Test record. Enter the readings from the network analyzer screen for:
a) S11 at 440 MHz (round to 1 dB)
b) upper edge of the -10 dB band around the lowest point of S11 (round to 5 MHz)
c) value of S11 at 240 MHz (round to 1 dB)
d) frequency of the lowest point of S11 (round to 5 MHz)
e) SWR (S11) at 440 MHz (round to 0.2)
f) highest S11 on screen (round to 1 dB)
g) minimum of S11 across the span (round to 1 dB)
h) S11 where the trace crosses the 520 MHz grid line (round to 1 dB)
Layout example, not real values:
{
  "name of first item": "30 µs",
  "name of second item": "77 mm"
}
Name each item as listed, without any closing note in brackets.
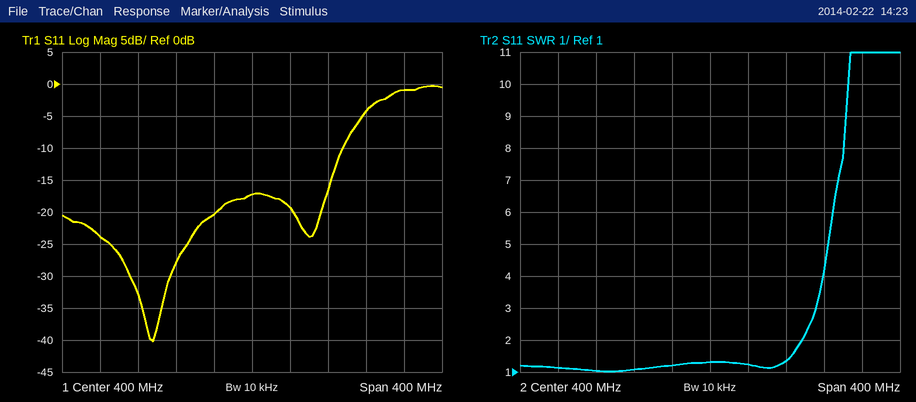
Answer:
{
  "S11 at 440 MHz": "-19 dB",
  "upper edge of the -10 dB band around the lowest point of S11": "495 MHz",
  "value of S11 at 240 MHz": "-24 dB",
  "frequency of the lowest point of S11": "295 MHz",
  "SWR (S11) at 440 MHz": "1.2",
  "highest S11 on screen": "0 dB",
  "minimum of S11 across the span": "-40 dB",
  "S11 where the trace crosses the 520 MHz grid line": "-4 dB"
}
